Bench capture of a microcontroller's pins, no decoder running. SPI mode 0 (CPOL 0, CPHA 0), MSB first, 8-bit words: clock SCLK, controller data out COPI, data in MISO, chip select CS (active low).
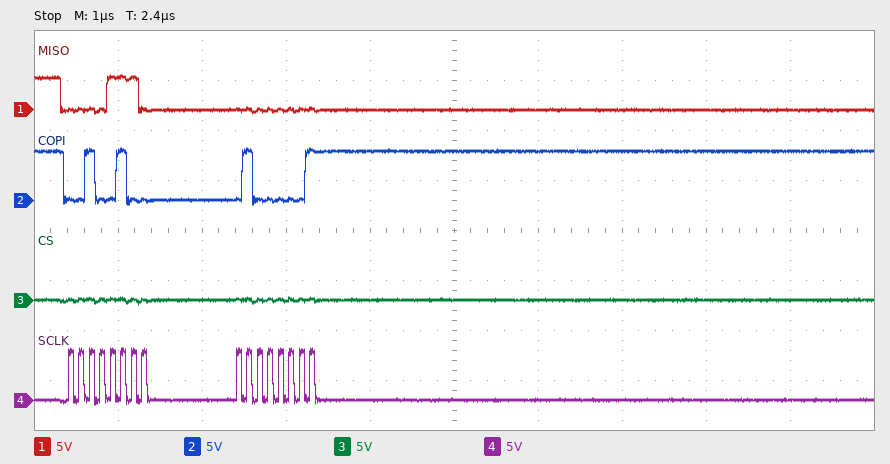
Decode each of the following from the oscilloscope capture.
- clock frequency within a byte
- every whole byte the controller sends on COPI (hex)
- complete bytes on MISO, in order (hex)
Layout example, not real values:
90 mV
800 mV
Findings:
8 MHz
24 41
0E 00
